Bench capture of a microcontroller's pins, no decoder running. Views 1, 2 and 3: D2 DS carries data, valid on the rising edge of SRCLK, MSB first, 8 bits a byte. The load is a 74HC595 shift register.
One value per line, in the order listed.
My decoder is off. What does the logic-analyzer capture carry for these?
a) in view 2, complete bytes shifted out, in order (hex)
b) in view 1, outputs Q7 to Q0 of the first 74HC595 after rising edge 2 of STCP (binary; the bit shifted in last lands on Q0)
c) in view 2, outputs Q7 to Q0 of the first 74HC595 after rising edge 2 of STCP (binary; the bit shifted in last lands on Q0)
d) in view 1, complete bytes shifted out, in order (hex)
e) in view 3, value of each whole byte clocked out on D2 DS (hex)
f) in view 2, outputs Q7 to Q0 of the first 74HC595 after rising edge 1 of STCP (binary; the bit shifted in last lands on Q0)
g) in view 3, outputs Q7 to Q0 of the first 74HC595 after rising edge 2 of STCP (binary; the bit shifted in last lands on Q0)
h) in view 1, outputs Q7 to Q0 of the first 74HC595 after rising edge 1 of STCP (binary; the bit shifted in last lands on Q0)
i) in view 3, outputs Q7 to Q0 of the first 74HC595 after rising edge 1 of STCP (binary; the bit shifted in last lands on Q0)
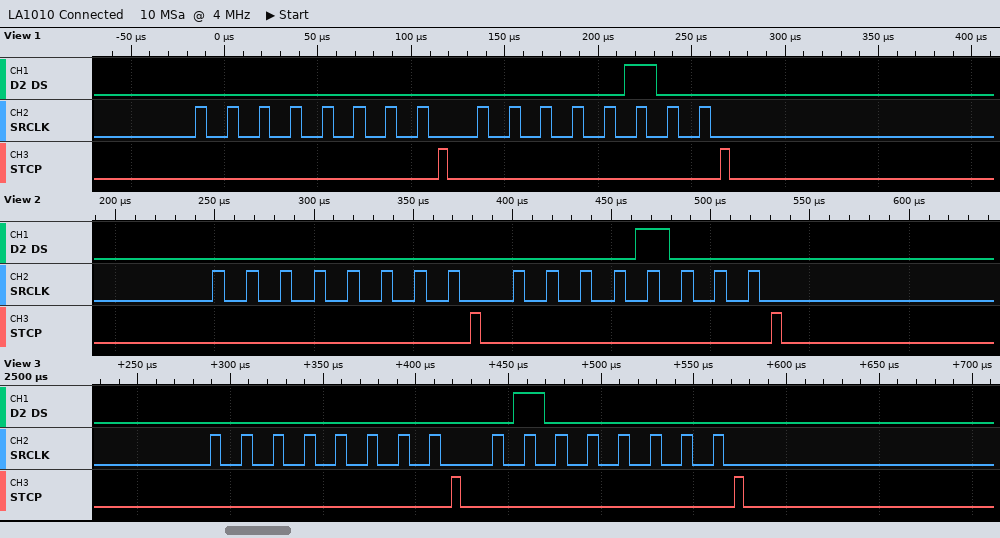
00 08
00000100
00001000
00 04
00 40
00000000
01000000
00000000
00000000
